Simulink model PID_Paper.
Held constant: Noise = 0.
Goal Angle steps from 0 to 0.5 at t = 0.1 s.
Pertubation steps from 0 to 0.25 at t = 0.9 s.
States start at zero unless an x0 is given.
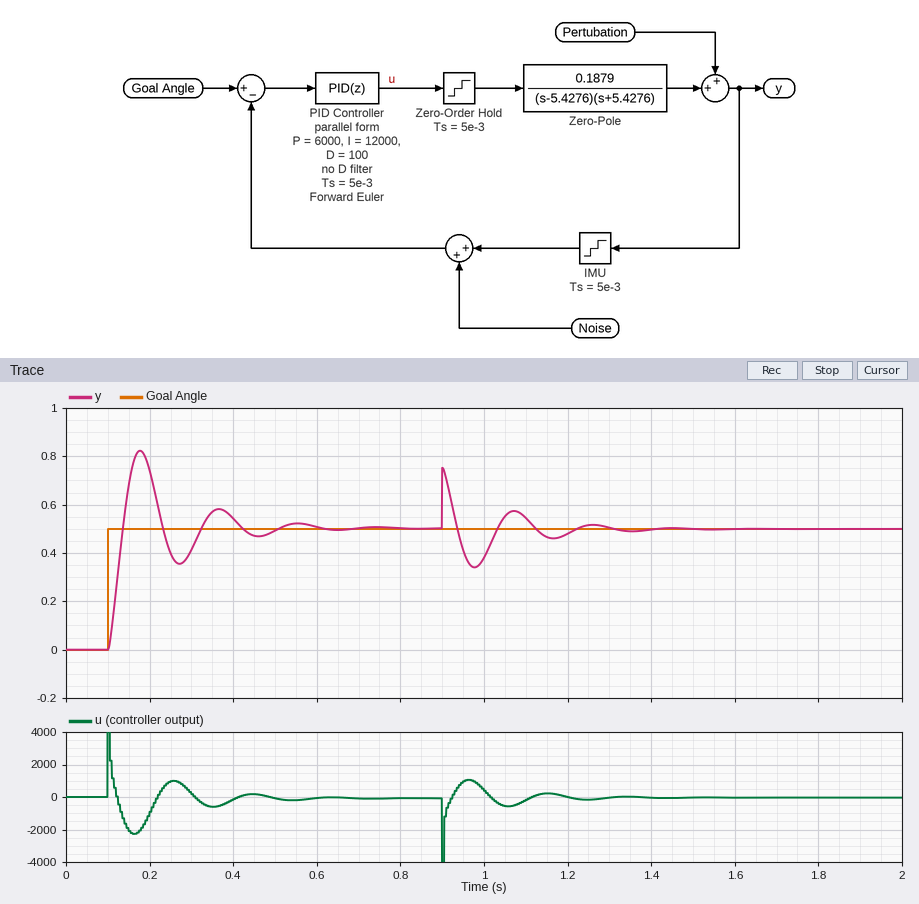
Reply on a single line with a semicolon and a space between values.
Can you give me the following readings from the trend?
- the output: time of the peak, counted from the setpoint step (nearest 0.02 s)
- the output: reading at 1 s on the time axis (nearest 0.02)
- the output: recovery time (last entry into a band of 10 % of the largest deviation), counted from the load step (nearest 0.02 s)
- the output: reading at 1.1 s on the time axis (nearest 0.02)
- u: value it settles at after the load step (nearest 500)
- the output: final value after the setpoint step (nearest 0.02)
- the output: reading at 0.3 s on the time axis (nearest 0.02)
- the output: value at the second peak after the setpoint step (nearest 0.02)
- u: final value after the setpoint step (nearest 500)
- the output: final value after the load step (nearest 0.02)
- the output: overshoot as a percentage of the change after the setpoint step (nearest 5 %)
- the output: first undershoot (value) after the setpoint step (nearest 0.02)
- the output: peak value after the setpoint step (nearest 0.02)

0.08 s; 0.38; 0.30 s; 0.54; 0; 0.50; 0.42; 0.58; 0; 0.50; 65 %; 0.36; 0.82
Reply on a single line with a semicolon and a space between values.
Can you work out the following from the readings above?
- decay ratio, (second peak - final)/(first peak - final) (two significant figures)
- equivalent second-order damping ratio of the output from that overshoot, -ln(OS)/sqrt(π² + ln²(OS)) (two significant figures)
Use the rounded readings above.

0.25; 0.14
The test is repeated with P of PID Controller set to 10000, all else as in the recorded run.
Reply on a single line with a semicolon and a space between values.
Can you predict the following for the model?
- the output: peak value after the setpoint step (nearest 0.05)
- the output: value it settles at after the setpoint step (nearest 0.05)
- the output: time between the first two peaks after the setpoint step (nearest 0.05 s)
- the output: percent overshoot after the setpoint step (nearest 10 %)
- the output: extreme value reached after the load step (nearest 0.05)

0.85; 0.50; 0.15 s; 70 %; 0.75
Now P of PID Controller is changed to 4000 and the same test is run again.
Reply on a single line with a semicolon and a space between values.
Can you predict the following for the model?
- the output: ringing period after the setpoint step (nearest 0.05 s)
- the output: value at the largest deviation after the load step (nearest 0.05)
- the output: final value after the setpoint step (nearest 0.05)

0.25 s; 0.75; 0.50
